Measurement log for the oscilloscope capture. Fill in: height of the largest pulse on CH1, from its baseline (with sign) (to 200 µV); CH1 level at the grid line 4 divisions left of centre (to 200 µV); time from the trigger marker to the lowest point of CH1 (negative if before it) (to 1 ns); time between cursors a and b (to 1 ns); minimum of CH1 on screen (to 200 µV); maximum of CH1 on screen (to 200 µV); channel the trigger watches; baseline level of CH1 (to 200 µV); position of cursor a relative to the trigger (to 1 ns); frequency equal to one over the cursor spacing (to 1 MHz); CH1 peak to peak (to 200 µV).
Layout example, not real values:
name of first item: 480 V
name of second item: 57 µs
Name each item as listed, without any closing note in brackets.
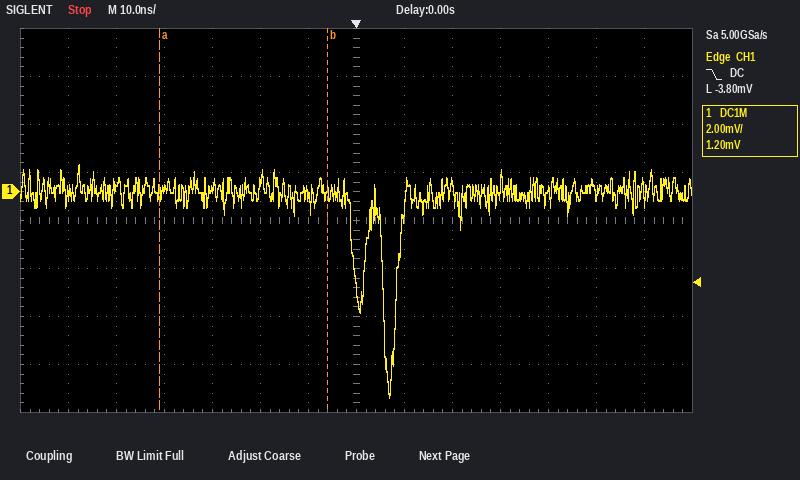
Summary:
height of the largest pulse on CH1, from its baseline (with sign): -8.6 mV
CH1 level at the grid line 4 divisions left of centre: 200 µV
time from the trigger marker to the lowest point of CH1 (negative if before it): +7 ns
time between cursors a and b: 35 ns
minimum of CH1 on screen: -8.6 mV
maximum of CH1 on screen: 1.2 mV
channel the trigger watches: CH1
baseline level of CH1: 0.0 mV
position of cursor a relative to the trigger: -41 ns
frequency equal to one over the cursor spacing: 29 MHz
CH1 peak to peak: 9.8 mV
